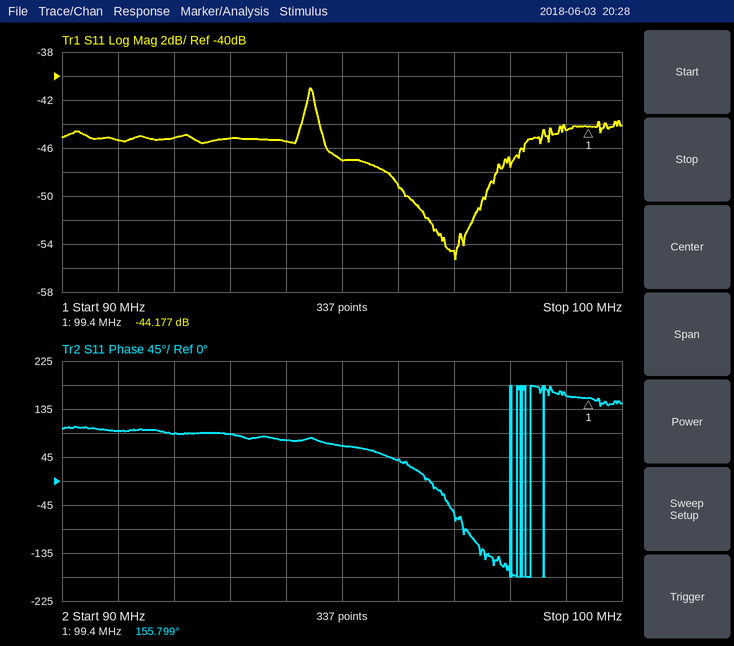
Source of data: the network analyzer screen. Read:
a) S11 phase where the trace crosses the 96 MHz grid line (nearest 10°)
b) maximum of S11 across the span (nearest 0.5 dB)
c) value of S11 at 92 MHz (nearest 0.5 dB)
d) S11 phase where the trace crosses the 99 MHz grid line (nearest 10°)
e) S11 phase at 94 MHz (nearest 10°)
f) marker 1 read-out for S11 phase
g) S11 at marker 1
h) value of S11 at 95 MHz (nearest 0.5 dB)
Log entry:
40°
-41.0 dB
-45.0 dB
160°
80°
155.799°
-44.177 dB
-47.0 dB
